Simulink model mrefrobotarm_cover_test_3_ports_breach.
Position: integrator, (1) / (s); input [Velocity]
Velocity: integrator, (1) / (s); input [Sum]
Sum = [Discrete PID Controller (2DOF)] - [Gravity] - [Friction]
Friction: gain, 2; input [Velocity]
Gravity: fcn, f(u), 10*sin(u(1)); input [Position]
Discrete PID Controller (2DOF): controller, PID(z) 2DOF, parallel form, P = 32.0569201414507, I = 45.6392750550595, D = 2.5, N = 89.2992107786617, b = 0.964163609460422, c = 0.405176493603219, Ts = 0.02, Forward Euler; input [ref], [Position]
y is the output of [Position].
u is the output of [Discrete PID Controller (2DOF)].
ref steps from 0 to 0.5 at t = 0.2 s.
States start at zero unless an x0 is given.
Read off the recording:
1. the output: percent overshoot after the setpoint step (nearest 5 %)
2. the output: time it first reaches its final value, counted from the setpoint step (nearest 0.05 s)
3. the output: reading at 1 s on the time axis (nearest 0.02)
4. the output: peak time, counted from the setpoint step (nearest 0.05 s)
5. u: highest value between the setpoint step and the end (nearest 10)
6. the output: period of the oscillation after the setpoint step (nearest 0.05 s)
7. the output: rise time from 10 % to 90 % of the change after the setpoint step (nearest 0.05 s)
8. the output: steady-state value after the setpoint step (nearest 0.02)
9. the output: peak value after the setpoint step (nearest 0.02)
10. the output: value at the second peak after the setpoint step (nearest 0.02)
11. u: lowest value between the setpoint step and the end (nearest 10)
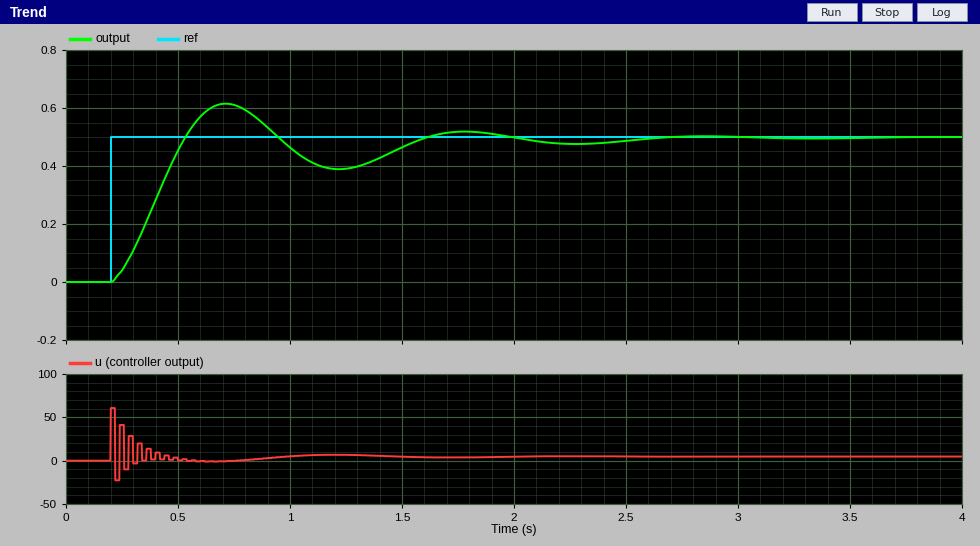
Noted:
25 %
0.35 s
0.46
0.50 s
60
1.05 s
0.25 s
0.50
0.62
0.52
-20
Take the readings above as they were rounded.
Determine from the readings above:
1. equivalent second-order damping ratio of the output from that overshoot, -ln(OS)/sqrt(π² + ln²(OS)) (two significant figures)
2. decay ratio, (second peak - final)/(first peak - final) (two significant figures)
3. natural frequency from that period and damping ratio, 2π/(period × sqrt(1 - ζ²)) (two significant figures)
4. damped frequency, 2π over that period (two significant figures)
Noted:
0.40
0.17
6.5 rad/s
6.0 rad/s
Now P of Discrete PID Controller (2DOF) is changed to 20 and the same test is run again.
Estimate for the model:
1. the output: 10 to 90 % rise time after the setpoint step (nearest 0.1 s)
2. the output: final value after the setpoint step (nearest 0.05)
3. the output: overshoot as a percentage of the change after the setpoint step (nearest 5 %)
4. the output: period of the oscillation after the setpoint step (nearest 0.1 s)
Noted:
0.3 s
0.50
20 %
1.3 s
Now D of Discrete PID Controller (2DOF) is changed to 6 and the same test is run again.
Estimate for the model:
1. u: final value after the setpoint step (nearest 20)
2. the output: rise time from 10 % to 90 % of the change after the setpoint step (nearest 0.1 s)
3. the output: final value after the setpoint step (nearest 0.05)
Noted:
0
0.3 s
0.50
